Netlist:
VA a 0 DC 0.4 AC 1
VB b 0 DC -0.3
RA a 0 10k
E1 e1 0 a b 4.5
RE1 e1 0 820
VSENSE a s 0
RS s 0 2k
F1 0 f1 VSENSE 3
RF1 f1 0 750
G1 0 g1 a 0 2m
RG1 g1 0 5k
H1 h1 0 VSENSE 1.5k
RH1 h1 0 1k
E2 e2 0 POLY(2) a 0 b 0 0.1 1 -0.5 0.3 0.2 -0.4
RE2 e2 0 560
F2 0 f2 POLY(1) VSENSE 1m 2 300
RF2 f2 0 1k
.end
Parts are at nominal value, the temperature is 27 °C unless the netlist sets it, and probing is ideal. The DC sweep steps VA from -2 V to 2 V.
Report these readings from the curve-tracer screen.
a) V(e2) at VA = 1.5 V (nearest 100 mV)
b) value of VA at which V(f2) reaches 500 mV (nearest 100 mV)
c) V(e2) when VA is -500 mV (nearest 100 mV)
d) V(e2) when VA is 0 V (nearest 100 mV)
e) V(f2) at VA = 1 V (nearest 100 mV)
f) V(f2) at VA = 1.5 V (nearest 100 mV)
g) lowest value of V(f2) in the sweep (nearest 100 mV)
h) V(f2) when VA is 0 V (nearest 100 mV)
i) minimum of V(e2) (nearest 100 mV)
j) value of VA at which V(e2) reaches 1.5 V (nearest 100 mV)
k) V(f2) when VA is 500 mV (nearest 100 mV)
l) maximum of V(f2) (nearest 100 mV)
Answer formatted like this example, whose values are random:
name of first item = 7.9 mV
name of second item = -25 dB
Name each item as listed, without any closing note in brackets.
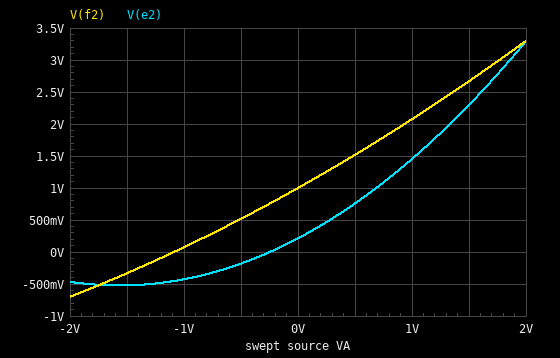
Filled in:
V(e2) at VA = 1.5 V = 2.3 V
value of VA at which V(f2) reaches 500 mV = -500 mV
V(e2) when VA is -500 mV = -200 mV
V(e2) when VA is 0 V = 200 mV
V(f2) at VA = 1 V = 2.1 V
V(f2) at VA = 1.5 V = 2.7 V
lowest value of V(f2) in the sweep = -700 mV
V(f2) when VA is 0 V = 1.0 V
minimum of V(e2) = -500 mV
value of VA at which V(e2) reaches 1.5 V = 1.0 V
V(f2) when VA is 500 mV = 1.5 V
maximum of V(f2) = 3.3 V
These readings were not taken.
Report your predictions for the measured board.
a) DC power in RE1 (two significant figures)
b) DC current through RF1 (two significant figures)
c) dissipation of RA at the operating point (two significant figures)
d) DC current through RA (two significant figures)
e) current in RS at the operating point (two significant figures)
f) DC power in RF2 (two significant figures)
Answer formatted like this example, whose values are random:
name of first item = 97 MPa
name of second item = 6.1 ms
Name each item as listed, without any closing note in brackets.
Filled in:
DC power in RE1 = 12 mW
DC current through RF1 = 600 µA
dissipation of RA at the operating point = 16 µW
DC current through RA = 40 µA
current in RS at the operating point = 200 µA
DC power in RF2 = 2.0 mW
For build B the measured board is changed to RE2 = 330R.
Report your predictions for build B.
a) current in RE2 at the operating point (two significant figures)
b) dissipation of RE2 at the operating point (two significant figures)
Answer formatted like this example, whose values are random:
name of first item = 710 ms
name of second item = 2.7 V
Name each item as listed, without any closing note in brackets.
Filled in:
current in RE2 at the operating point = 1.9 mA
dissipation of RE2 at the operating point = 1.2 mW
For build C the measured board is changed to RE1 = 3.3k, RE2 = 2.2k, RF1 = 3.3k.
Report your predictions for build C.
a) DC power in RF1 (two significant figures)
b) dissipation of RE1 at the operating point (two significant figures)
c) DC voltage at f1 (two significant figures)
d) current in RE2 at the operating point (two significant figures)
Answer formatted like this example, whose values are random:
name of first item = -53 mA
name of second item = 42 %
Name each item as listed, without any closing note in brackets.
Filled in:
DC power in RF1 = 1.2 mW
dissipation of RE1 at the operating point = 3.0 mW
DC voltage at f1 = 2.0 V
current in RE2 at the operating point = 290 µA
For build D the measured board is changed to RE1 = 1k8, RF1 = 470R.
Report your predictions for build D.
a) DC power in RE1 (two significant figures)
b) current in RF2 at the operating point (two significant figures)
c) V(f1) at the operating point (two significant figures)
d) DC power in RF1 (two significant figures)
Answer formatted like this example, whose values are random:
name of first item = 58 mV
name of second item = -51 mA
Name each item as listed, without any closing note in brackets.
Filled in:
DC power in RE1 = 5.5 mW
current in RF2 at the operating point = 1.4 mA
V(f1) at the operating point = 280 mV
DC power in RF1 = 170 µW
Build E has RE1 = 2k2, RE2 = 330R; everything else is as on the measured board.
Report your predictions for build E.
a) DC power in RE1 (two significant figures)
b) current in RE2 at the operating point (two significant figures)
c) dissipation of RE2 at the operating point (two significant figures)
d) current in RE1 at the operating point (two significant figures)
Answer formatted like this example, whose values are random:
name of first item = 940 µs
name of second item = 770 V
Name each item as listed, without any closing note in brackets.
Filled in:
DC power in RE1 = 4.5 mW
current in RE2 at the operating point = 1.9 mA
dissipation of RE2 at the operating point = 1.2 mW
current in RE1 at the operating point = 1.4 mA
